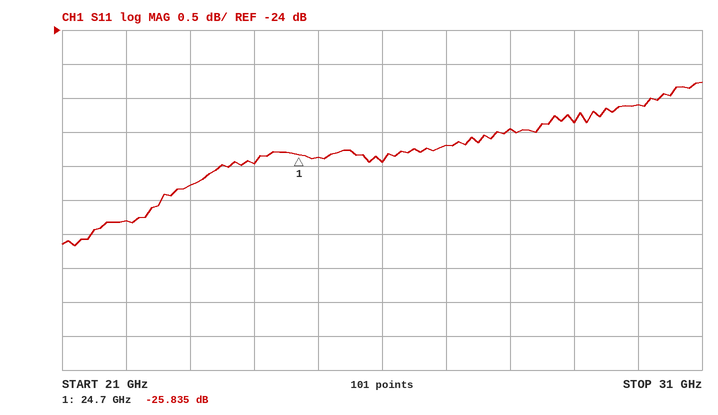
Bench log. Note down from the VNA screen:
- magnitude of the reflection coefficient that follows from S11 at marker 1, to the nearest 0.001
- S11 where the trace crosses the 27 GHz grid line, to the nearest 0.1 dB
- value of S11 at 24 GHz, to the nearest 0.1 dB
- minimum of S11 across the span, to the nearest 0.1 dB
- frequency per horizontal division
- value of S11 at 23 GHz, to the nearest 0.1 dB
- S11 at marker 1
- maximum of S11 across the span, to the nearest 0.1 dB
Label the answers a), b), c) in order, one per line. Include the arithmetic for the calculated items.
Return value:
a) 10^(-25.835/20) ≈ 0.051
b) -25.7 dB
c) -26.0 dB
d) -27.2 dB
e) 1 GHz
f) -26.3 dB
g) -25.835 dB
h) -24.8 dB
